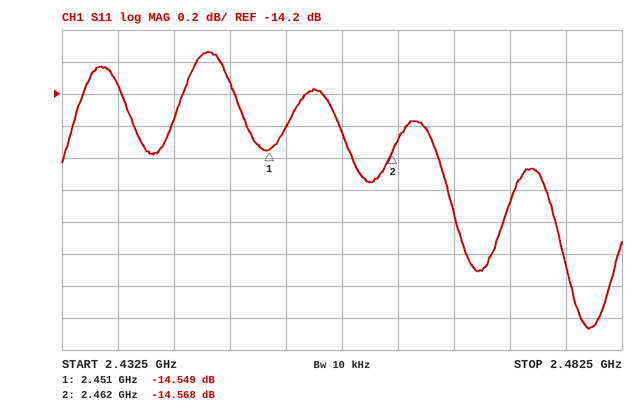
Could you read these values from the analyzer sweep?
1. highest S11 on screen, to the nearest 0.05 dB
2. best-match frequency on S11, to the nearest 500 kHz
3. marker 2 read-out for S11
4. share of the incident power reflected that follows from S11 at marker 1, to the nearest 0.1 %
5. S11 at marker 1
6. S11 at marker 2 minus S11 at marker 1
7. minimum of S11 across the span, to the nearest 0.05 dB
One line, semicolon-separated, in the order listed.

-13.95 dB; 2.4795 GHz; -14.568 dB; 3.5 %; -14.549 dB; -0.019 dB; -15.65 dB
